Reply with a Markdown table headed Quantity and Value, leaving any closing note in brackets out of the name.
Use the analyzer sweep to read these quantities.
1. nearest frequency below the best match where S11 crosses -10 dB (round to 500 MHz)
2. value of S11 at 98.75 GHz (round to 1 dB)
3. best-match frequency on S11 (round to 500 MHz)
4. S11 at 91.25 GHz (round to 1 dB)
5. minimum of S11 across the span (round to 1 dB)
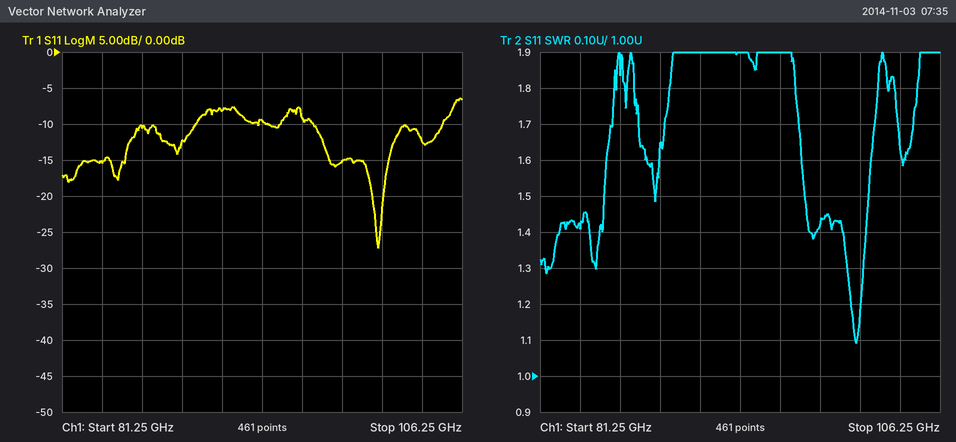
| Quantity | Value |
|---|---|
| nearest frequency below the best match where S11 crosses -10 dB | 97.0 GHz |
| value of S11 at 98.75 GHz | -15 dB |
| best-match frequency on S11 | 101.0 GHz |
| S11 at 91.25 GHz | -8 dB |
| minimum of S11 across the span | -27 dB |
